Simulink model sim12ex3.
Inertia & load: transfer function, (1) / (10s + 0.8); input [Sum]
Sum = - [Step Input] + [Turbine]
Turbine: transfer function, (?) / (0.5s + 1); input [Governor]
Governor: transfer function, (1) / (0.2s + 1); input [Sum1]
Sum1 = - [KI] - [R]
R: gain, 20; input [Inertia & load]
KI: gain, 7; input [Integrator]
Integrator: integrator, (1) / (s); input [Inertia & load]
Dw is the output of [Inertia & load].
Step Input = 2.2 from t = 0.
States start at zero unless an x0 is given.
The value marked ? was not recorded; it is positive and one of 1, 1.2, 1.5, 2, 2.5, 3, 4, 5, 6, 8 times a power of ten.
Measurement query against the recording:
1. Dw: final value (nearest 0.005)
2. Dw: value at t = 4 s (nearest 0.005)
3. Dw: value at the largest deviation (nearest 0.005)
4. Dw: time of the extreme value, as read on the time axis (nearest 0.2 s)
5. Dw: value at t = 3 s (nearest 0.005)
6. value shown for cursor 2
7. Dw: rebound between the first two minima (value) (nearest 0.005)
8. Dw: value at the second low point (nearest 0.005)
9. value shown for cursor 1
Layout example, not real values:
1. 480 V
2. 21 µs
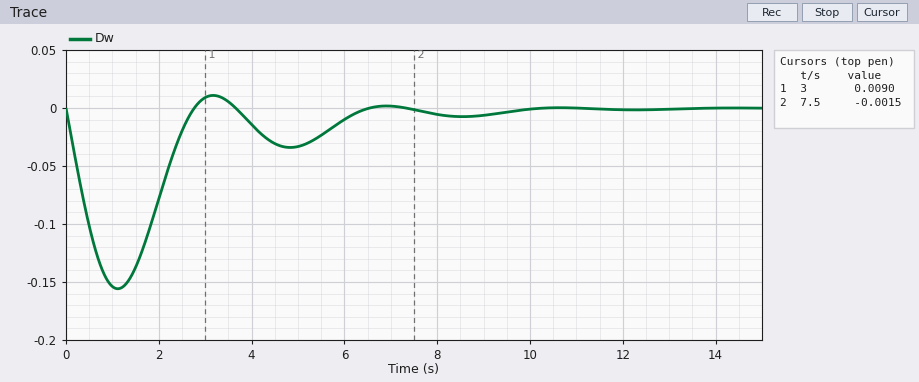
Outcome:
1. 0.000
2. -0.015
3. -0.155
4. 1.2 s
5. 0.010
6. -0.0015
7. 0.010
8. -0.035
9. 0.0090
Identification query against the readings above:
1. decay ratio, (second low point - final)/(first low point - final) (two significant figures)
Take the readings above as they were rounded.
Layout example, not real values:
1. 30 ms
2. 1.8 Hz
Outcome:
1. 0.23
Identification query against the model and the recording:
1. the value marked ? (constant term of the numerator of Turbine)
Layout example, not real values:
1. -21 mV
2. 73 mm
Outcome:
1. 1
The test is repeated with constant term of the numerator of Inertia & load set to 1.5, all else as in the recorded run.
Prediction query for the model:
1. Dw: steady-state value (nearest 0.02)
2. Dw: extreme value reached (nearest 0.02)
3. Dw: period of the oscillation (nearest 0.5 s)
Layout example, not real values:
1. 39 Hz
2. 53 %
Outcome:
1. 0.00
2. -0.20
3. 3.0 s
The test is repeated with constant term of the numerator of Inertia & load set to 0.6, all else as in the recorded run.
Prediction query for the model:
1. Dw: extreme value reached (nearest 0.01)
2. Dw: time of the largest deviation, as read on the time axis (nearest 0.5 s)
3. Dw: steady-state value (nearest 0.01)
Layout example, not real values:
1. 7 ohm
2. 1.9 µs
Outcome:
1. -0.12
2. 1.5 s
3. 0.00
